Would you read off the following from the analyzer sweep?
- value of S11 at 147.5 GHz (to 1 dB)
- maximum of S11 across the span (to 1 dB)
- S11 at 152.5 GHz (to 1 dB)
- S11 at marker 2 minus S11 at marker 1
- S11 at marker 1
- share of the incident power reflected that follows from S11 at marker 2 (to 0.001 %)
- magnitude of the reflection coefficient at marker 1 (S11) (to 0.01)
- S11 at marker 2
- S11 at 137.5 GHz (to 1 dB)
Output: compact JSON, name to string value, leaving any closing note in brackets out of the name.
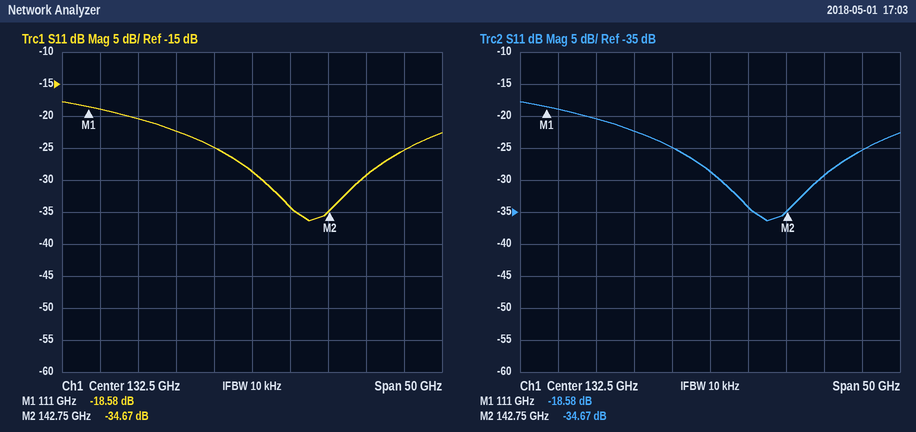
{"value of S11 at 147.5 GHz": "-29 dB", "maximum of S11 across the span": "-18 dB", "S11 at 152.5 GHz": "-25 dB", "S11 at marker 2 minus S11 at marker 1": "-16.09 dB", "S11 at marker 1": "-18.58 dB", "share of the incident power reflected that follows from S11 at marker 2": "0.034 %", "magnitude of the reflection coefficient at marker 1 (S11)": "0.12", "S11 at marker 2": "-34.67 dB", "S11 at 137.5 GHz": "-34 dB"}
